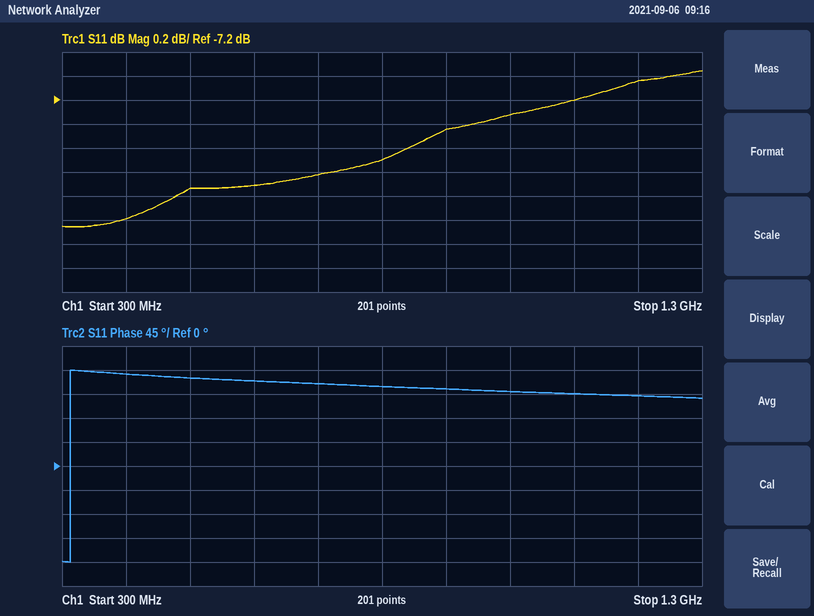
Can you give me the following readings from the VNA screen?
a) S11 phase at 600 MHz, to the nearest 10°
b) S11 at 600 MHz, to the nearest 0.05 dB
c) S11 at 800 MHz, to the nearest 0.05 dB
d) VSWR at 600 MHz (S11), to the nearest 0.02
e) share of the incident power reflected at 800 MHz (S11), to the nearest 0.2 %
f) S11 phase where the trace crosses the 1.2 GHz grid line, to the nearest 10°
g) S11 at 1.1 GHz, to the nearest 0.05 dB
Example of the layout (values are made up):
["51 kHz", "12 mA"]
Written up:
["160°", "-7.90 dB", "-7.70 dB", "2.34", "17.0 %", "130°", "-7.20 dB"]
